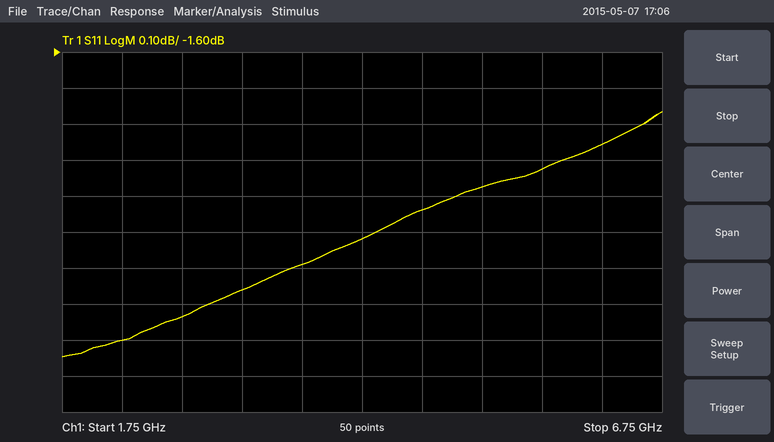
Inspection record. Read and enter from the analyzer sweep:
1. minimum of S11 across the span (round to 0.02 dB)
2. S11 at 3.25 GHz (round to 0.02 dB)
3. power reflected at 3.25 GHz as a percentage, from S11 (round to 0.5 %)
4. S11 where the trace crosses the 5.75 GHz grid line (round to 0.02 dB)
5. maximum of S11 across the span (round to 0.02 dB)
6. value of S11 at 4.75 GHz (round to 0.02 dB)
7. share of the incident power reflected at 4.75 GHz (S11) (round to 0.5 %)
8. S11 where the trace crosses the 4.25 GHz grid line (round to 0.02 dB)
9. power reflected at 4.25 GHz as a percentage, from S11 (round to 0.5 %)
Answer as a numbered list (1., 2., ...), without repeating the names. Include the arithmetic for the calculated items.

1. -2.44 dB
2. -2.26 dB
3. 10^(-2.26/10) ≈ 59.4 %, so 59.5 % to the nearest 0.5 %
4. -1.92 dB
5. -1.76 dB
6. -2.04 dB
7. 10^(-2.04/10) ≈ 62.5 %
8. -2.12 dB
9. 10^(-2.12/10) ≈ 61.4 %, so 61.5 % to the nearest 0.5 %
